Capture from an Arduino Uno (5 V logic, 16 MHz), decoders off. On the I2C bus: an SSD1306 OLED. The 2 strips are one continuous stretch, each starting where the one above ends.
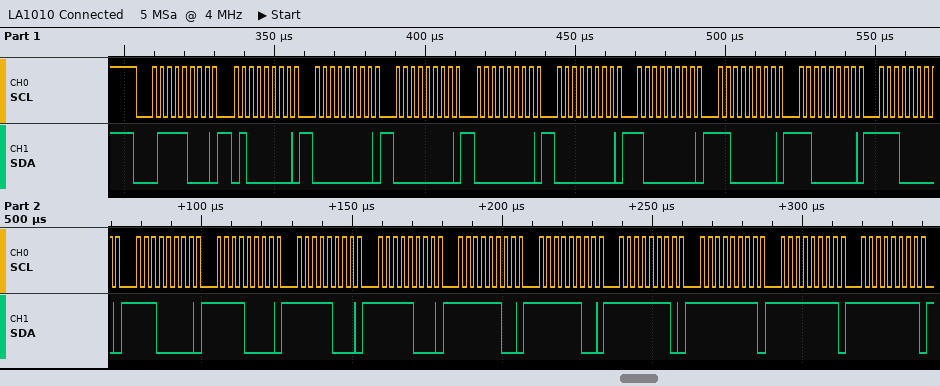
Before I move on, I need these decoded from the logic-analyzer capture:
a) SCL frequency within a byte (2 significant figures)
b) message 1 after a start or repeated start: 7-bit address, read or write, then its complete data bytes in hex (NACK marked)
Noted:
400 kHz
0x3C write: 40 00 00 00 00 80 C0 C0 E0 E0 F0 F8 F8 FC FC FE FF FF FF
